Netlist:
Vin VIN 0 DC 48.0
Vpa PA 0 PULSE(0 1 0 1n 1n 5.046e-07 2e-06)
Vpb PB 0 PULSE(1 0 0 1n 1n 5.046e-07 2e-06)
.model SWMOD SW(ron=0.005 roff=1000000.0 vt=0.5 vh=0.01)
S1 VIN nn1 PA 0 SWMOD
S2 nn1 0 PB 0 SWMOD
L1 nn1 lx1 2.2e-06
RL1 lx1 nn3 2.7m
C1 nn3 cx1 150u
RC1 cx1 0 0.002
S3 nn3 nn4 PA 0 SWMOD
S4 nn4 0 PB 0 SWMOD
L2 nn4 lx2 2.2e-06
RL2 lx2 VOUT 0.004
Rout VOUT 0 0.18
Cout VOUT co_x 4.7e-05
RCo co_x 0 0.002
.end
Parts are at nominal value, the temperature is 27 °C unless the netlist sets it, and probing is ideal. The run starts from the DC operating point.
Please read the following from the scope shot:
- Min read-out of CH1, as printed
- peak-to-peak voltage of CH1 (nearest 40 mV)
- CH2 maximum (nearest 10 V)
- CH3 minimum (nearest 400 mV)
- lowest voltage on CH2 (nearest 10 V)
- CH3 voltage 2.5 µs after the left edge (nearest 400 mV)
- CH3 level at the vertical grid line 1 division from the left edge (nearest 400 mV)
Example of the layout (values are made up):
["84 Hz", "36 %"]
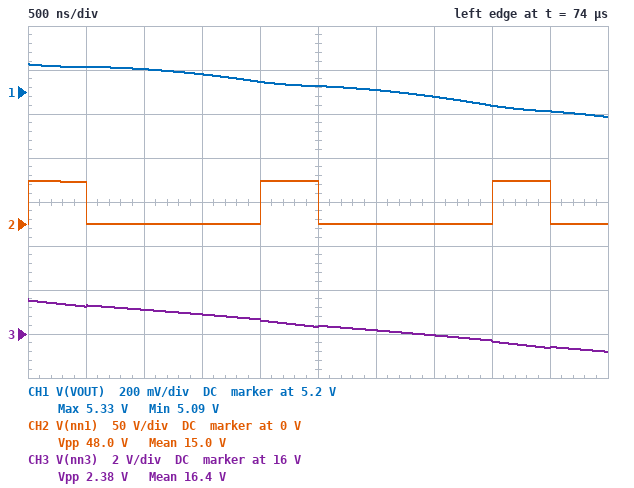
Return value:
["5.09 V", "240 mV", "50 V", "15.2 V", "0 V", "16.4 V", "17.2 V"]
